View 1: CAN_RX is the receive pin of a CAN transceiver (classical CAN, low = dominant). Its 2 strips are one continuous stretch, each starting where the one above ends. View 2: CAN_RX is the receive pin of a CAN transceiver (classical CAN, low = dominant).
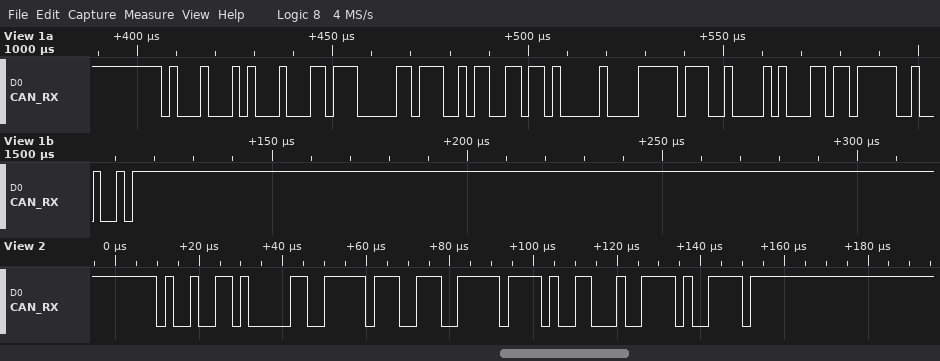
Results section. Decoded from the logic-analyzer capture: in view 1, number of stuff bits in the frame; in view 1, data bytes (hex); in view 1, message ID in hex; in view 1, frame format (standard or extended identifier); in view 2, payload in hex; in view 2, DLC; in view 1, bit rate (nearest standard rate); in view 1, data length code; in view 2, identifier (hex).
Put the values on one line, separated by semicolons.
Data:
4; DC 17 2C DA 00 FF 21 46; 0x445; standard; FF 39 FF 4C; 4; 500 kbit/s; 8; 0x49A
